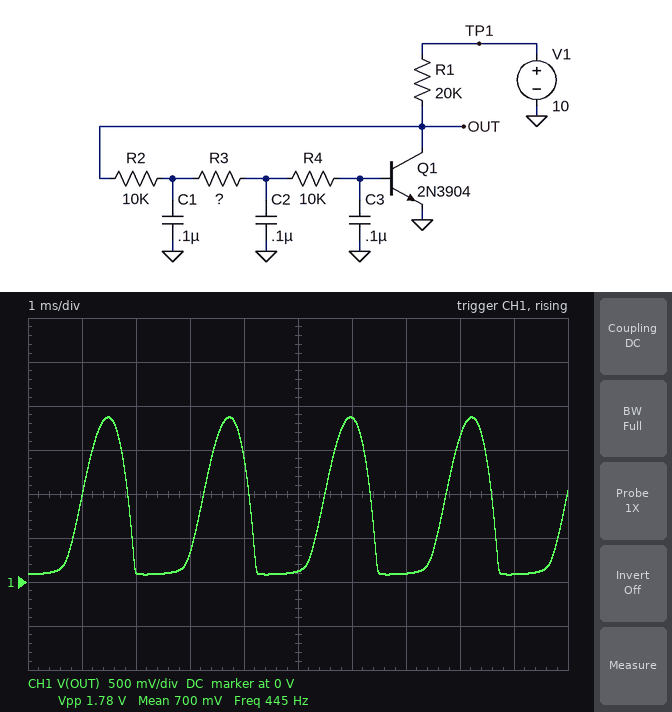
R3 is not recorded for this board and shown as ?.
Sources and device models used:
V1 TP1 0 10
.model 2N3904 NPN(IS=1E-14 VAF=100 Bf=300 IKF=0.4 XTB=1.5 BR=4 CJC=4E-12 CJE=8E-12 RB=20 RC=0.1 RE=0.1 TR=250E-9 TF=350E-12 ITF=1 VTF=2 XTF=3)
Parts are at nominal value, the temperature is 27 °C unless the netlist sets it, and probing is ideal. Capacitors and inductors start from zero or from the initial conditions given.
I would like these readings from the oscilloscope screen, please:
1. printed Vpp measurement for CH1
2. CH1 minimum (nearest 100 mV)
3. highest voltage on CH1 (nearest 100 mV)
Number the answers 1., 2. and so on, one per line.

1. 1.78 V
2. 100 mV
3. 1.9 V
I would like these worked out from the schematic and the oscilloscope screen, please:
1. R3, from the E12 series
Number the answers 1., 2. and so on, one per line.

1. 18 kΩ
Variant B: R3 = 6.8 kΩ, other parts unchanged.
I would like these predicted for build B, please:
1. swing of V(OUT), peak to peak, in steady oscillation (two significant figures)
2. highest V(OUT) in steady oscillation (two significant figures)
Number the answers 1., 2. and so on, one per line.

1. 1.6 V
2. 1.7 V
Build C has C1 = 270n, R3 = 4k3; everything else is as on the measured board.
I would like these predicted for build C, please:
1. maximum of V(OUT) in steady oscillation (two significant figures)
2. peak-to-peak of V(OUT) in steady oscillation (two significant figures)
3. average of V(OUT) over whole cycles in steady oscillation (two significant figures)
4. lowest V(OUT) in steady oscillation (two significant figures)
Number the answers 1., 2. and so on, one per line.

1. 1.5 V
2. 1.4 V
3. 690 mV
4. 99 mV
